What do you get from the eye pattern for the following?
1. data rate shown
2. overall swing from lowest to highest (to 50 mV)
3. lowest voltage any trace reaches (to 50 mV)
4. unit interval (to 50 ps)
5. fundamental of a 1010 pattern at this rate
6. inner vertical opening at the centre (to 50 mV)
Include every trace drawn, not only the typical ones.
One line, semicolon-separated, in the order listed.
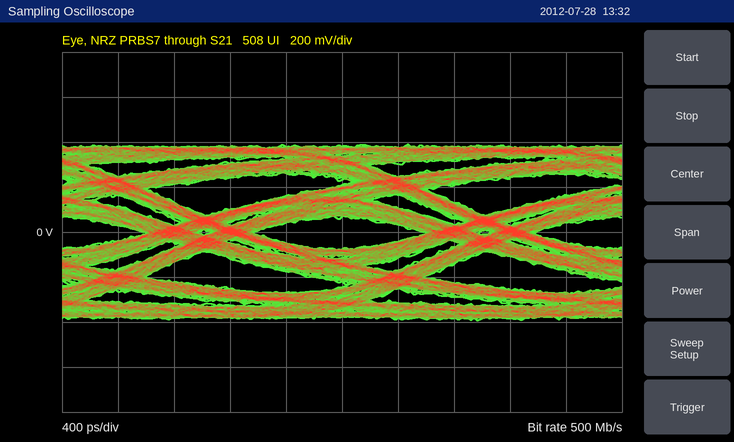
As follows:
500 Mb/s; 800 mV; -400 mV; 2.00 ns; 250 MHz; 150 mV
